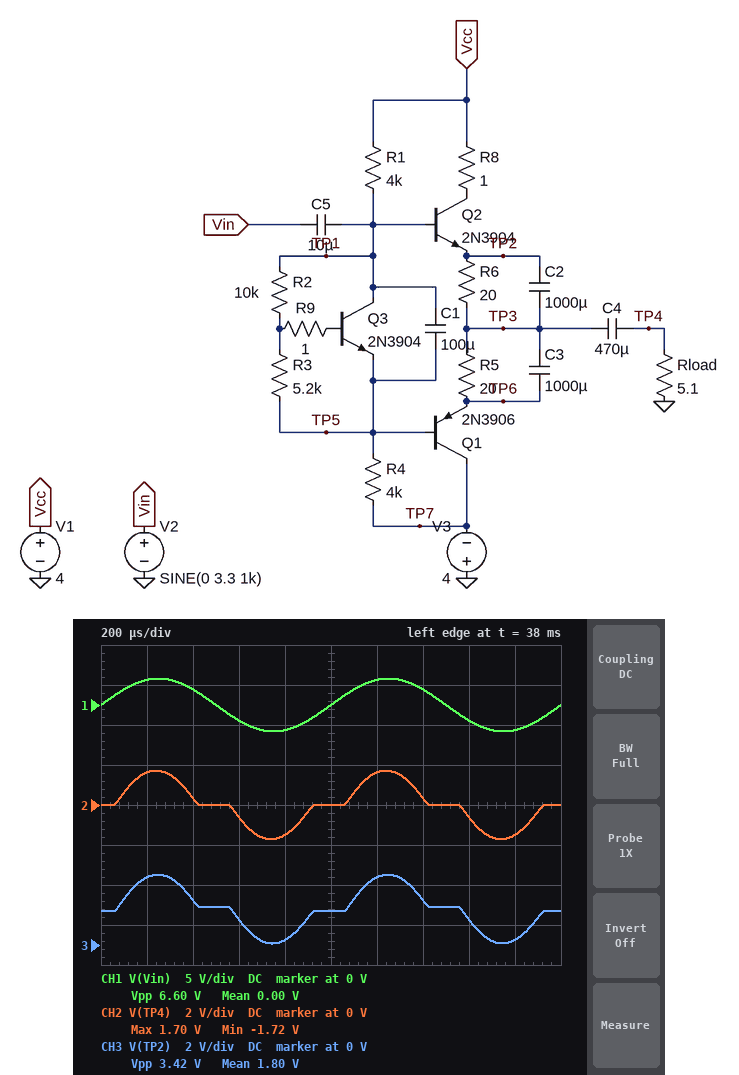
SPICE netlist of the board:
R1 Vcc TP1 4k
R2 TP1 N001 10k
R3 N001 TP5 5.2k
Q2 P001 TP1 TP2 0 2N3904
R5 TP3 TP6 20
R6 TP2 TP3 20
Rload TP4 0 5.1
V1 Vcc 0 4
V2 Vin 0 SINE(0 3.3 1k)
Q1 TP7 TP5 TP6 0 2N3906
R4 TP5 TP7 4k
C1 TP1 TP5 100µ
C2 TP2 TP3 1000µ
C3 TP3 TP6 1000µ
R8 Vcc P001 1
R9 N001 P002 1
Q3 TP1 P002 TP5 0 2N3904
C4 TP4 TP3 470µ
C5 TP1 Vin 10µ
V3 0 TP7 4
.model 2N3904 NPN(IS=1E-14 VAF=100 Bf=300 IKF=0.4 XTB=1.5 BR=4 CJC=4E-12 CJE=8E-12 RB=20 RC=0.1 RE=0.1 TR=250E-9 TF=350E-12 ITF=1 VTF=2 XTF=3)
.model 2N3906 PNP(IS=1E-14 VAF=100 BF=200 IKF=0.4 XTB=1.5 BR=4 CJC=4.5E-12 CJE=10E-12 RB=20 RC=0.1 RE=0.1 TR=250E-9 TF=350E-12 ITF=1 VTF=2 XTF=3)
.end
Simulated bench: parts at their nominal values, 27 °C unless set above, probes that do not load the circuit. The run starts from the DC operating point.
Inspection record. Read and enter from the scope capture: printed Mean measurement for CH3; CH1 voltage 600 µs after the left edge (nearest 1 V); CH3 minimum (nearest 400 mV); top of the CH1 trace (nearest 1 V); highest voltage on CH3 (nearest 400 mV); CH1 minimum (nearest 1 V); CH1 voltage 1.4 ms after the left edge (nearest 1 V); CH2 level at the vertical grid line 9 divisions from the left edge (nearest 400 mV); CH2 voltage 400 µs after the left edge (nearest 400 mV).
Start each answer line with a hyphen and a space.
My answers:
- 1.80 V
- -2 V
- 0 V
- 3 V
- 3.6 V
- -3 V
- 2 V
- -1.6 V
- 400 mV
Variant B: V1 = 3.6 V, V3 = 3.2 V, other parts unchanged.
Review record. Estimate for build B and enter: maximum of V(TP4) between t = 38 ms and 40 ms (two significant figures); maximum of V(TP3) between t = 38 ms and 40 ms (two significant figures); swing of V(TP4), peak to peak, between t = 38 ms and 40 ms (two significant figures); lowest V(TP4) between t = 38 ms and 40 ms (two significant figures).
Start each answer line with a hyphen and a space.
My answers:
- 1.6 V
- 1.7 V
- 3.2 V
- -1.6 V
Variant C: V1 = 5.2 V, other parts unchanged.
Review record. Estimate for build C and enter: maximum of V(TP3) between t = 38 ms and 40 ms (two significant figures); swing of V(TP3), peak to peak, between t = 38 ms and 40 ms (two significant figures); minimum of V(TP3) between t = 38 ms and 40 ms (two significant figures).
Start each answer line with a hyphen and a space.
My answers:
- 2.7 V
- 3.5 V
- -760 mV
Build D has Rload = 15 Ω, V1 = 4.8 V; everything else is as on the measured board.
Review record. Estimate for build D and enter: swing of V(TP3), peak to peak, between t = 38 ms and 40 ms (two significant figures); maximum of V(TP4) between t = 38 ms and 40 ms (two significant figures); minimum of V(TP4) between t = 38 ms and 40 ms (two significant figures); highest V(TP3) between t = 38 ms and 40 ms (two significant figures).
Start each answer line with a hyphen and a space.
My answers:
- 5.0 V
- 2.5 V
- -2.5 V
- 3.1 V
